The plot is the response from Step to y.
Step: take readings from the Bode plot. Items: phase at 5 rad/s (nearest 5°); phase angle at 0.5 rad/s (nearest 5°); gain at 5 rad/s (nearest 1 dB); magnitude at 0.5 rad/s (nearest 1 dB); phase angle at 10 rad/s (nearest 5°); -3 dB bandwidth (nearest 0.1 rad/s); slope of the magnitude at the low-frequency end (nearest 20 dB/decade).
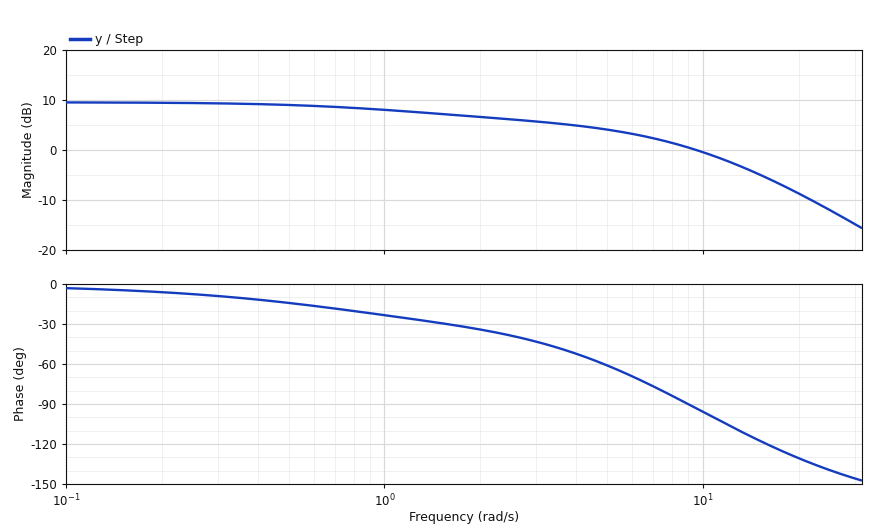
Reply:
-60°
-15°
4 dB
9 dB
-95°
2.1 rad/s
0 dB/decade
